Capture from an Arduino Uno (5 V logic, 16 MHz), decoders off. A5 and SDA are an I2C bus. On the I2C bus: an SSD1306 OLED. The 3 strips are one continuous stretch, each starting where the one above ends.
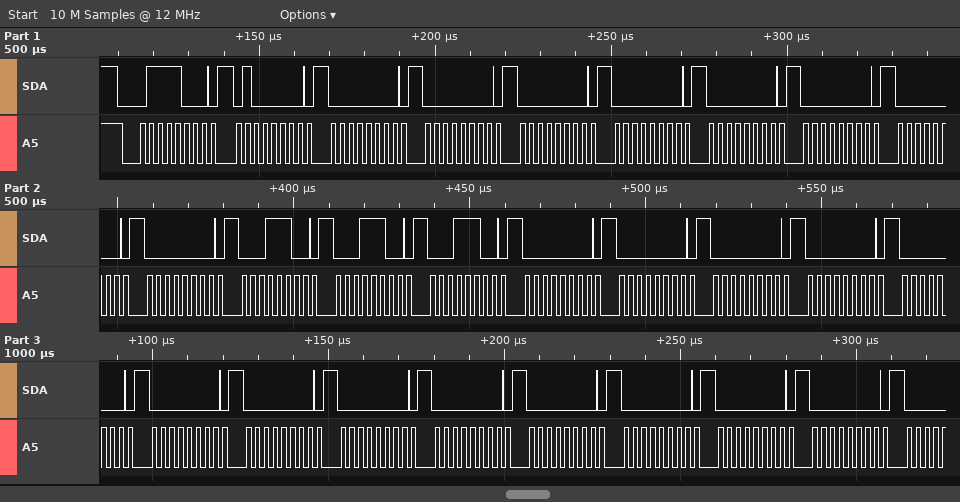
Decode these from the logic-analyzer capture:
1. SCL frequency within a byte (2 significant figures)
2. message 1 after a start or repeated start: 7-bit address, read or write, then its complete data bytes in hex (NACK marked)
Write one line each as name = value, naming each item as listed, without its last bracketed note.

SCL frequency within a byte = 400 kHz
message 1 after a start or repeated start: 7-bit address, read or write, then its complete data bytes in hex = 0x3C write: 40 00 00 00 00 00 00 00 00 1C 1C 1C 00 00 00 00 00 00 00 00 00 00 00 00 00
